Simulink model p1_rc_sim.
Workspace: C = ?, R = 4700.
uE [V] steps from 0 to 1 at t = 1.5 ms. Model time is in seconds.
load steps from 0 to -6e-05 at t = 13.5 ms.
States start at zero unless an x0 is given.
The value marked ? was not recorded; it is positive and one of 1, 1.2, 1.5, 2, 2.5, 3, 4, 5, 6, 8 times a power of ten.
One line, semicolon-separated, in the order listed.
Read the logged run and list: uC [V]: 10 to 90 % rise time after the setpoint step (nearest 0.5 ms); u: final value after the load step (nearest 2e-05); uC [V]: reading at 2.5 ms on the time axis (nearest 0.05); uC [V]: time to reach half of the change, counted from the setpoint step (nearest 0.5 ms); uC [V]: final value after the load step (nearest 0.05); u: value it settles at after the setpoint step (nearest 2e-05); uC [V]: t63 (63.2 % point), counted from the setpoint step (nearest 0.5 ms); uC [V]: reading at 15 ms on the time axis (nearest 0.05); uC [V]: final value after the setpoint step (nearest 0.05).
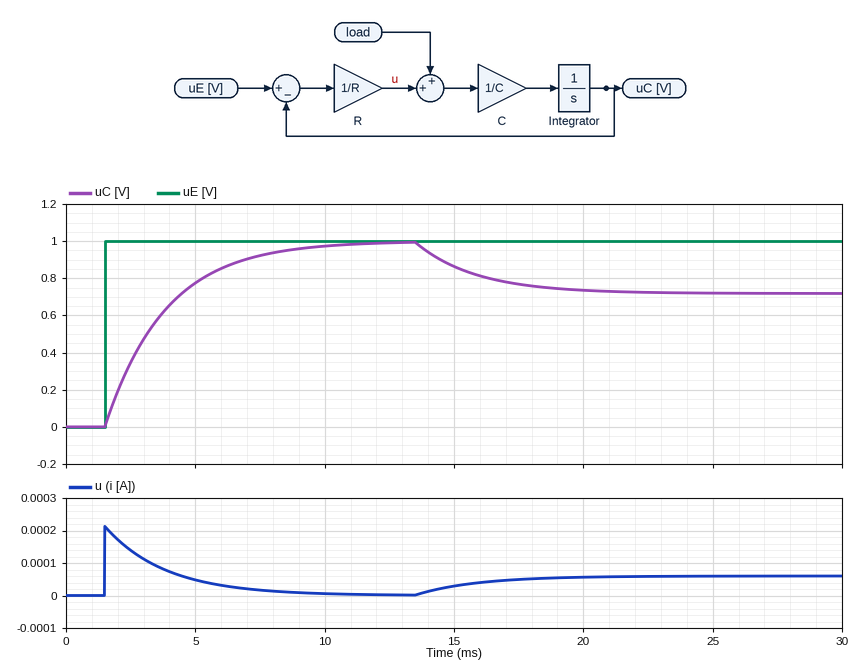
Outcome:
5.0 ms; 0.00006; 0.35; 1.5 ms; 0.70; 0.00000; 2.5 ms; 0.85; 1.00
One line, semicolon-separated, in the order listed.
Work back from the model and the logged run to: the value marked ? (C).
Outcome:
5e-07
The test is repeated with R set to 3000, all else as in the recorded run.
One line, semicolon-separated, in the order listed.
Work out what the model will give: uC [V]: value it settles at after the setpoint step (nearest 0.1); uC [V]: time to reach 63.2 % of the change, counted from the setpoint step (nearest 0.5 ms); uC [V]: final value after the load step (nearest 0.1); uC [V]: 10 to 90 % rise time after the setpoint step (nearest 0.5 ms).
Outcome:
1.0; 1.5 ms; 0.8; 3.5 ms
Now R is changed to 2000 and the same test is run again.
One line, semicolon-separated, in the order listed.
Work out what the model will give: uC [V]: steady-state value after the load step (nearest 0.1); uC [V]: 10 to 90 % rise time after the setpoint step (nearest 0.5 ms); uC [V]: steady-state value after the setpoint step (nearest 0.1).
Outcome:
0.9; 2.0 ms; 1.0
